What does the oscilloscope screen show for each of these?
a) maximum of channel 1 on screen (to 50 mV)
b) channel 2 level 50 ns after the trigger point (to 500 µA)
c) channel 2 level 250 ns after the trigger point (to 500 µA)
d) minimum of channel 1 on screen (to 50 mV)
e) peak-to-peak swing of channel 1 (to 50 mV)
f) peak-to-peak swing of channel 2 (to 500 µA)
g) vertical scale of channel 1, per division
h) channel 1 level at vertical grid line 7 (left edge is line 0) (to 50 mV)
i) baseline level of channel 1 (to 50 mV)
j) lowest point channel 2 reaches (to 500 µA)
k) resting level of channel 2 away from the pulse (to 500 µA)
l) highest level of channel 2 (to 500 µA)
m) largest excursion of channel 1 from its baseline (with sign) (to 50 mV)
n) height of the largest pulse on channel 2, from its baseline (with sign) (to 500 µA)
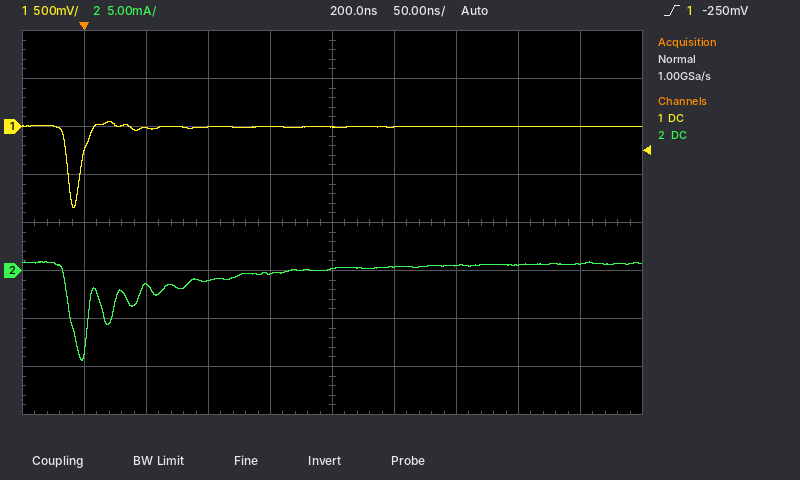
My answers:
50 mV
-1.5 mA
500 µA
-850 mV
900 mV
10.5 mA
500 mV
0 mV
0 mV
-9.5 mA
500 µA
1.0 mA
-850 mV
-10.0 mA
